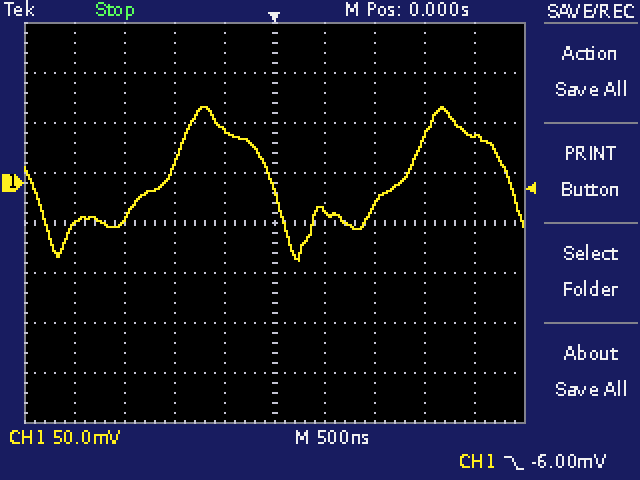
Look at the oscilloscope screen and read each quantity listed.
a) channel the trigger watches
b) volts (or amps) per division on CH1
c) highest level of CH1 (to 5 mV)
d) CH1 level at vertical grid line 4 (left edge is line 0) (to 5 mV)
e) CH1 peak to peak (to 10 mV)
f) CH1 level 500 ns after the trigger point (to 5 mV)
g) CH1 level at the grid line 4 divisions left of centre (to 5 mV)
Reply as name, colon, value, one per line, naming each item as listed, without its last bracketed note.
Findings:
channel the trigger watches: CH1
volts (or amps) per division on CH1: 50 mV
highest level of CH1: 75 mV
CH1 level at vertical grid line 4 (left edge is line 0): 55 mV
CH1 peak to peak: 150 mV
CH1 level 500 ns after the trigger point: -30 mV
CH1 level at the grid line 4 divisions left of centre: -40 mV
